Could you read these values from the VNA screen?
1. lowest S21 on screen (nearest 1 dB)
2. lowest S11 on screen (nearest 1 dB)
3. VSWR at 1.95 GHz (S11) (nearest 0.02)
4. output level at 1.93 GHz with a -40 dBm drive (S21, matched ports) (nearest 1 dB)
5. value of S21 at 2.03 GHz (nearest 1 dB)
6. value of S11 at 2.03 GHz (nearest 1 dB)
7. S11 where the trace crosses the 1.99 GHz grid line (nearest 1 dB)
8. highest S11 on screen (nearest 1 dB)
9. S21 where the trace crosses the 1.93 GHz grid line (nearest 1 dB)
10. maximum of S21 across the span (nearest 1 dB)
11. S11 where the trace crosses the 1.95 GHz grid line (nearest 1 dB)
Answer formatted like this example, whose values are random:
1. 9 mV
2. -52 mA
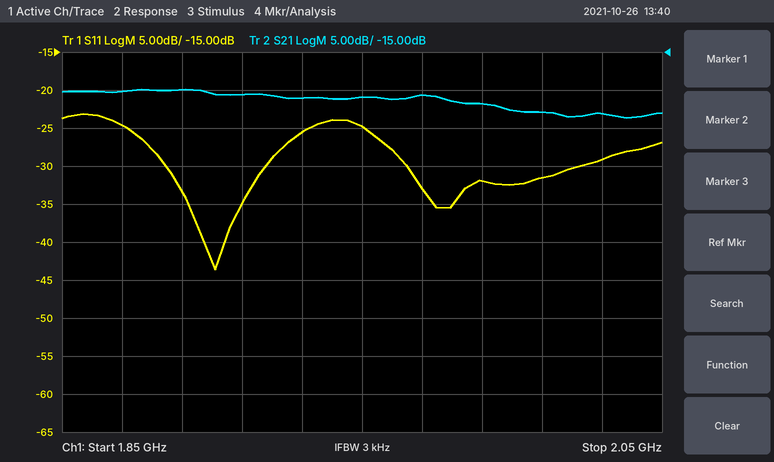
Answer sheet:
1. -24 dB
2. -44 dB
3. 1.12
4. -61 dBm
5. -23 dB
6. -29 dB
7. -32 dB
8. -23 dB
9. -21 dB
10. -20 dB
11. -25 dB
